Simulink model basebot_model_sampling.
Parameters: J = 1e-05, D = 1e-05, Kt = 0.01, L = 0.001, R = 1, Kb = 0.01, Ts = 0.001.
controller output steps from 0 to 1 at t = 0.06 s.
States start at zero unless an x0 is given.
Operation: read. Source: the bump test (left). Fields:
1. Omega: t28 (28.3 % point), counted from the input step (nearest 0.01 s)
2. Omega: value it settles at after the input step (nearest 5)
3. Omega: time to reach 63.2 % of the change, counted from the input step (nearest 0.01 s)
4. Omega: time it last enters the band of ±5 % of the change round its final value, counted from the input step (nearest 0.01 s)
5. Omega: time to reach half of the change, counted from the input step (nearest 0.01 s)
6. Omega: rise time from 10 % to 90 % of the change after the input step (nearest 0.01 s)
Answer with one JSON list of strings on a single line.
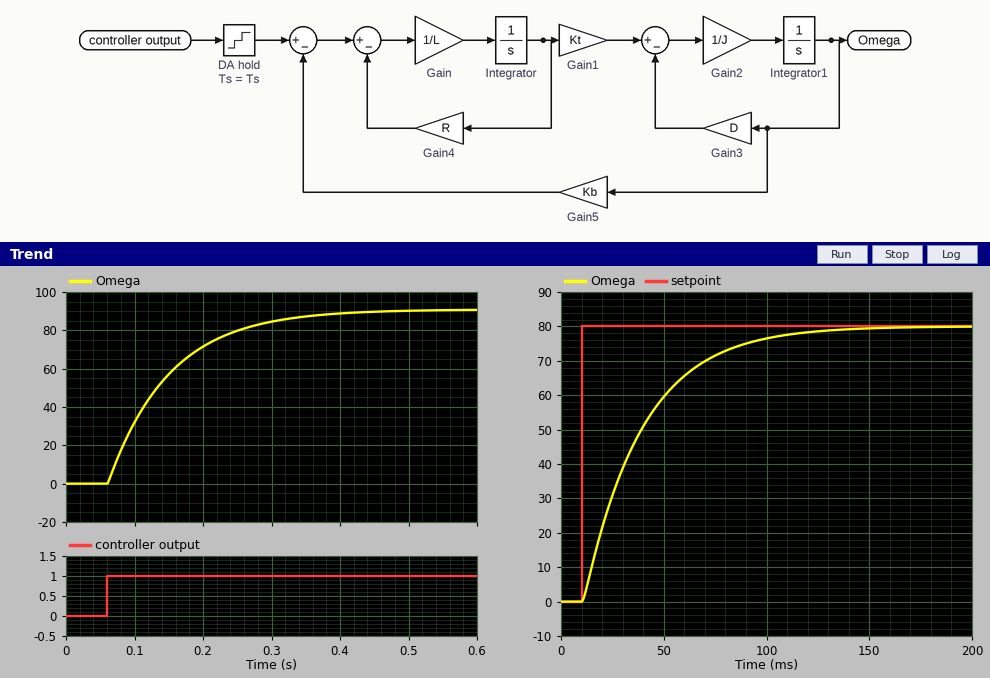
["0.03 s", "90", "0.09 s", "0.27 s", "0.06 s", "0.20 s"]
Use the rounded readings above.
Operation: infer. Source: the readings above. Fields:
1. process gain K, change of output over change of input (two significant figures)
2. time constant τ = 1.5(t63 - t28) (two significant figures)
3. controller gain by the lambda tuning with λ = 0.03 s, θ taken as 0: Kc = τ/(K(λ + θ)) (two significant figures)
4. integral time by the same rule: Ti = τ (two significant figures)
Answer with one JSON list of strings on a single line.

["90", "0.090 s", "0.033", "0.090 s"]
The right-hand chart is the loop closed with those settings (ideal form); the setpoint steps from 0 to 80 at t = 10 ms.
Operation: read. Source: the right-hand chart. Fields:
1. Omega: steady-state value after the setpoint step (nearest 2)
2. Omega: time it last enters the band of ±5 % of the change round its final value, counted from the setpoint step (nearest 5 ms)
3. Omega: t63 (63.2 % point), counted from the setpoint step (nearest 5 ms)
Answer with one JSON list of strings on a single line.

["80", "85 ms", "30 ms"]
